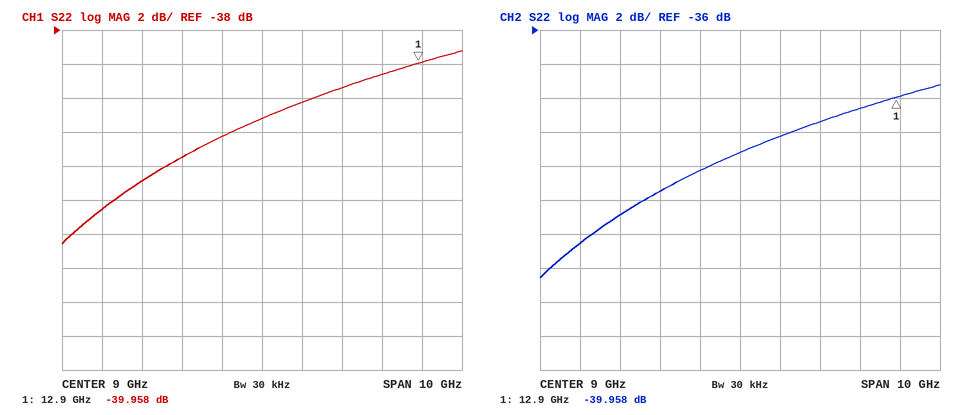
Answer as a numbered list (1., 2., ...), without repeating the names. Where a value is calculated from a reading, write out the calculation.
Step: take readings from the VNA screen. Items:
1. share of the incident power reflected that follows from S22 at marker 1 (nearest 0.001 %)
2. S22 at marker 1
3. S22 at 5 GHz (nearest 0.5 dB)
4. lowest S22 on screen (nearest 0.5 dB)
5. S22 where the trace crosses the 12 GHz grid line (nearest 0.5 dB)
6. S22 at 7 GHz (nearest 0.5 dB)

1. 10^(-39.958/10) ≈ 0.010 %
2. -39.958 dB
3. -48.5 dB
4. -50.5 dB
5. -40.5 dB
6. -45.5 dB
